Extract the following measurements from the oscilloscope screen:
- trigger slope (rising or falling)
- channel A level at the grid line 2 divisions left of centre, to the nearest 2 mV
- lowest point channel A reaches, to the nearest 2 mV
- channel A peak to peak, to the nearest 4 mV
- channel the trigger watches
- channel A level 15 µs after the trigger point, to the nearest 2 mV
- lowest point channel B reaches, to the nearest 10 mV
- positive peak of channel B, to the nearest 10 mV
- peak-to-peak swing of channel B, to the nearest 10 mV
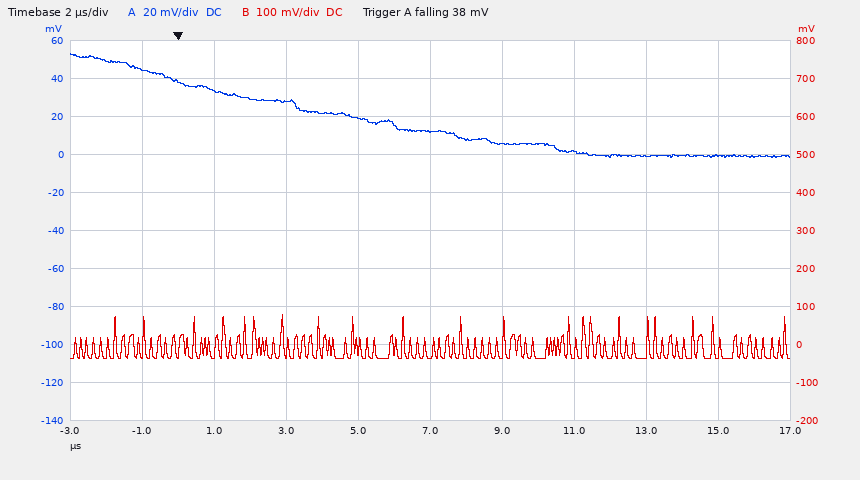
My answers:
falling
28 mV
-2 mV
56 mV
channel A
0 mV
-40 mV
80 mV
120 mV
